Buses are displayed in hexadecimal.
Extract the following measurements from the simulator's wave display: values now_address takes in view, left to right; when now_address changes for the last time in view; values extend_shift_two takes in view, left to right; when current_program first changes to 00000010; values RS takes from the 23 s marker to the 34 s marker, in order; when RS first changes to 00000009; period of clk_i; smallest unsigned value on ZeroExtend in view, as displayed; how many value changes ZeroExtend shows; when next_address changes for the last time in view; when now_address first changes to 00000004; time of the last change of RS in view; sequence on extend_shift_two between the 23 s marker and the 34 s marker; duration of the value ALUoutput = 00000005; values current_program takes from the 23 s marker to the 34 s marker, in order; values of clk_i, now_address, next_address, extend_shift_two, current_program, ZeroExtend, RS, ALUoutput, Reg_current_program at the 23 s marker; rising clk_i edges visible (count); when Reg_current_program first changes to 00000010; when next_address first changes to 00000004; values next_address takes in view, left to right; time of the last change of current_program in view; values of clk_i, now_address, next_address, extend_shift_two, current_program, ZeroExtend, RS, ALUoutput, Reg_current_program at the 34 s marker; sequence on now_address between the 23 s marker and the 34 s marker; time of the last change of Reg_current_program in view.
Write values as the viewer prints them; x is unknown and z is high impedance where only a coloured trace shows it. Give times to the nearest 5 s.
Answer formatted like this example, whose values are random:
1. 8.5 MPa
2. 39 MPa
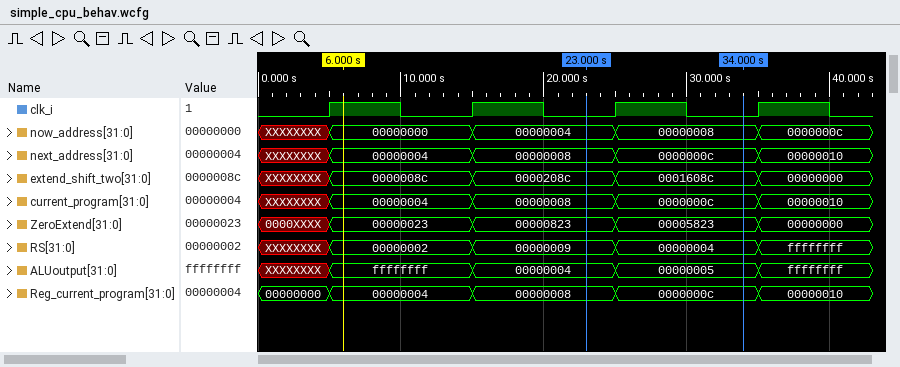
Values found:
1. XXXXXXXX, 00000000, 00000004, 00000008, 0000000c
2. 35 s
3. XXXXXXXX, 0000008c, 0000208c, 0001608c, 00000000
4. 35 s
5. 00000009, 00000004
6. 15 s
7. 10 s
8. 00000000
9. 4
10. 35 s
11. 15 s
12. 35 s
13. 0000208c, 0001608c
14. 10 s
15. 00000008, 0000000c
16. clk_i=0, now_address=00000004, next_address=00000008, extend_shift_two=0000208c, current_program=00000008, ZeroExtend=00000823, RS=00000009, ALUoutput=00000004, Reg_current_program=00000008
17. 4
18. 35 s
19. 5 s
20. XXXXXXXX, 00000004, 00000008, 0000000c, 00000010
21. 35 s
22. clk_i=0, now_address=00000008, next_address=0000000c, extend_shift_two=0001608c, current_program=0000000c, ZeroExtend=00005823, RS=00000004, ALUoutput=00000005, Reg_current_program=0000000c
23. 00000004, 00000008
24. 35 s
